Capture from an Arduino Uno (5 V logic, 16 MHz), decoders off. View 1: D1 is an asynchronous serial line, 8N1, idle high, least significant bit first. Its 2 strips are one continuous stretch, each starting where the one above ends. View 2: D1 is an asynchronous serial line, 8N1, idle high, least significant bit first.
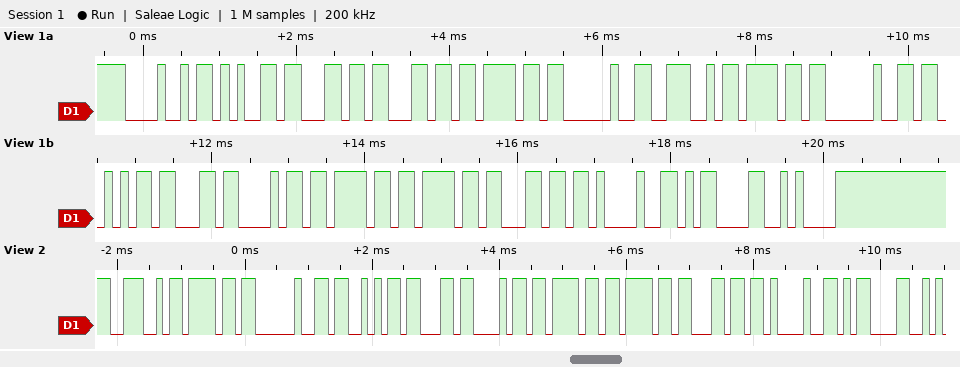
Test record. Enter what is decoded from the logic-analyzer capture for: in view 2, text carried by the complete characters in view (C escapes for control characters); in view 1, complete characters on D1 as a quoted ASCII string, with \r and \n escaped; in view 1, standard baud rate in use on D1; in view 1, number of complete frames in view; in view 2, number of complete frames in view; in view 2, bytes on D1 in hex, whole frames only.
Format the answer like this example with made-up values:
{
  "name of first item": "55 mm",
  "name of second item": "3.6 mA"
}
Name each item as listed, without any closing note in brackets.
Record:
{
  "in view 2, text carried by the complete characters in view": "\"No School!\\r\"",
  "in view 1, complete characters on D1 as a quoted ASCII string, with \\r and \\n escaped": "\"Hello No School!\\r\\n\"",
  "in view 1, standard baud rate in use on D1": "9600 baud",
  "in view 1, number of complete frames in view": "18",
  "in view 2, number of complete frames in view": "11",
  "in view 2, bytes on D1 in hex, whole frames only": "0x4E 0x6F 0x20 0x53 0x63 0x68 0x6F 0x6F 0x6C 0x21 0x0D"
}
